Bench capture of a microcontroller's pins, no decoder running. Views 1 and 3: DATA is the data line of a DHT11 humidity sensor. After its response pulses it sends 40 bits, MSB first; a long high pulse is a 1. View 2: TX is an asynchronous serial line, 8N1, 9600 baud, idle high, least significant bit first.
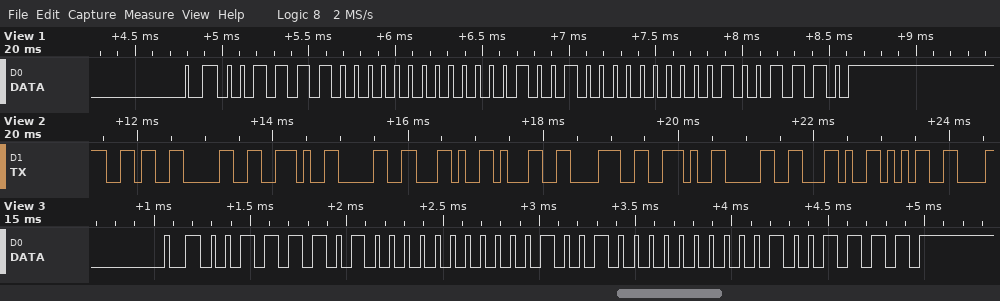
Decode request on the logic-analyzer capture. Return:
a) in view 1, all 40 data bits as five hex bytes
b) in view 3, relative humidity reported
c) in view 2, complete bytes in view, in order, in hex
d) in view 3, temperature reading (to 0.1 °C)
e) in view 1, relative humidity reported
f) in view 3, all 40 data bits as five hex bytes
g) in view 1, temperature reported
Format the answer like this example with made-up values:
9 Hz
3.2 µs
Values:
3C 00 12 00 4E
61 %
0x36 0x30 0x2E 0x30 0x2C 0x31 0x38 0x2E 0x30 0x2C 0x35
18.0 °C
60 %
3D 00 12 00 4F
18.0 °C
